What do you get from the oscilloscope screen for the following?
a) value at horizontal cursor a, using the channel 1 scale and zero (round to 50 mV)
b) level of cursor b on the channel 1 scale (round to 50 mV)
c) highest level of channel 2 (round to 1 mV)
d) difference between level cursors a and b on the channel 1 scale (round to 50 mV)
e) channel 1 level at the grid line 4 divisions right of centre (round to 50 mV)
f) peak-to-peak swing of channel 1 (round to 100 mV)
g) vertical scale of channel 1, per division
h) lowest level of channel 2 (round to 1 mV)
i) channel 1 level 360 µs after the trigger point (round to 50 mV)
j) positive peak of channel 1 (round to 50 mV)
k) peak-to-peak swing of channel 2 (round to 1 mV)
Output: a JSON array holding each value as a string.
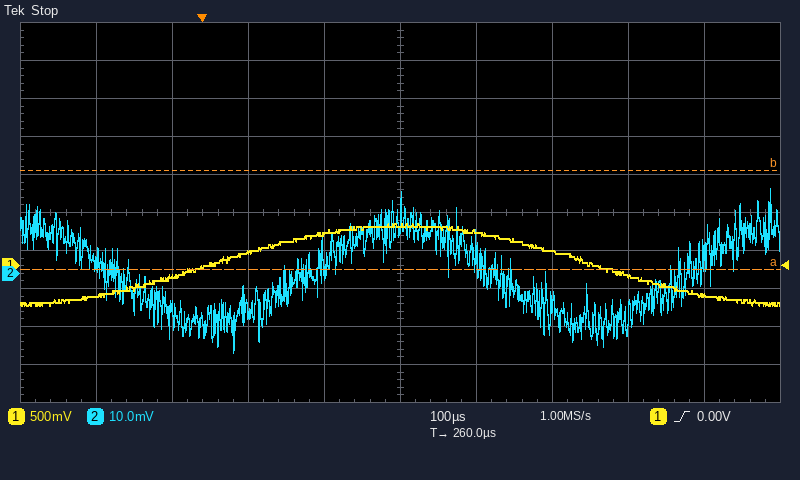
["-50 mV", "1.25 V", "22 mV", "1.30 V", "-400 mV", "1.10 V", "500 mV", "-21 mV", "450 mV", "550 mV", "43 mV"]
